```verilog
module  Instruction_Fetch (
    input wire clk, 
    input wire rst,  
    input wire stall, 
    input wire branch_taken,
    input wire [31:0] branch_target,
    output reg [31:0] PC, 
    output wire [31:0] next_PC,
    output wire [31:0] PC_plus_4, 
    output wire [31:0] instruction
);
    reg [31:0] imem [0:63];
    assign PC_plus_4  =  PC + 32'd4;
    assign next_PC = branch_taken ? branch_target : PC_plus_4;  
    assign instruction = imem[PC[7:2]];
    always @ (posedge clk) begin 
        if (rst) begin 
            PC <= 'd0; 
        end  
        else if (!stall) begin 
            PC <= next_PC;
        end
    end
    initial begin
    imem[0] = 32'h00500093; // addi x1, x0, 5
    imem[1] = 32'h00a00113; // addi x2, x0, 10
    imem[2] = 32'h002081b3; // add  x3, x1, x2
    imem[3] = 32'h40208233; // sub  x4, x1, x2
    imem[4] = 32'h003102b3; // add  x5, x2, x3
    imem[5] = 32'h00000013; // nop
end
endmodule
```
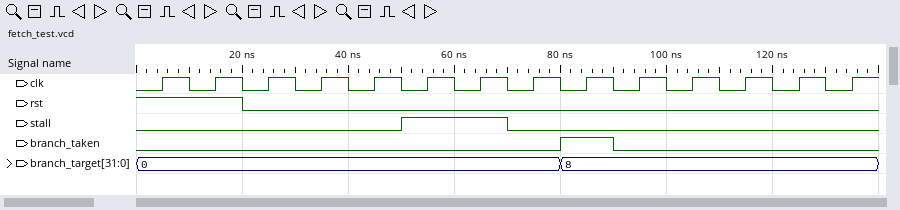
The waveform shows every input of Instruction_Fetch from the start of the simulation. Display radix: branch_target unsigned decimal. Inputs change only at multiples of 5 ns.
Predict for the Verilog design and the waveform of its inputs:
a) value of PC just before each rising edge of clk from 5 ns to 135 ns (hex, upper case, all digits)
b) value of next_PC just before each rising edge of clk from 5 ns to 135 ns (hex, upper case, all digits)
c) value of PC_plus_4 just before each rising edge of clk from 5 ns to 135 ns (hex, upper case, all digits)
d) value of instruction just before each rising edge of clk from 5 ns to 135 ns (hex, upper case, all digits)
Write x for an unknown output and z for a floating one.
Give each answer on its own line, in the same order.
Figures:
x, 00000000, 00000000, 00000004, 00000008, 0000000C, 0000000C, 0000000C, 00000010, 00000008, 0000000C, 00000010, 00000014, 00000018
x, 00000004, 00000004, 00000008, 0000000C, 00000010, 00000010, 00000010, 00000008, 0000000C, 00000010, 00000014, 00000018, 0000001C
x, 00000004, 00000004, 00000008, 0000000C, 00000010, 00000010, 00000010, 00000014, 0000000C, 00000010, 00000014, 00000018, 0000001C
x, 00500093, 00500093, 00A00113, 002081B3, 40208233, 40208233, 40208233, 003102B3, 002081B3, 40208233, 003102B3, 00000013, x
